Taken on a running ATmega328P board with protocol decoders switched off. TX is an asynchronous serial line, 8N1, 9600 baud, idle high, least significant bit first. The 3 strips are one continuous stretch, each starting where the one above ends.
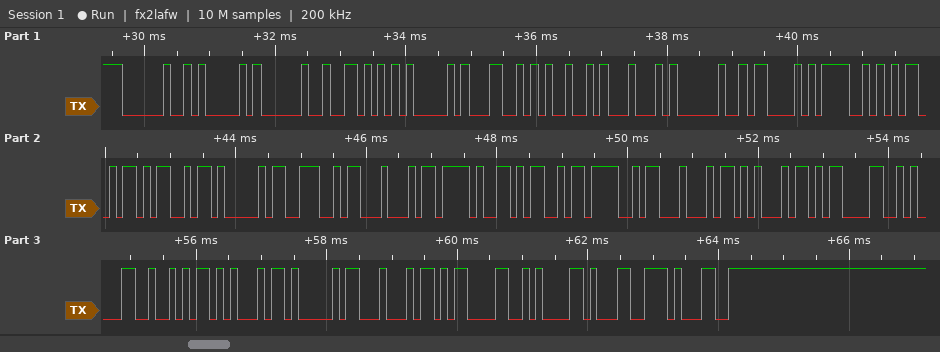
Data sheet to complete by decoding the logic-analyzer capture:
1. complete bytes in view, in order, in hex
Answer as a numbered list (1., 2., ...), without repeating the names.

1. 20 41 20 56 41 4C 49 44 20 43 4F 4D 4D 41 4E 44 2F 4D 4F 44 45 0D 0A 52 45 41 44 0D 0A 31 31
